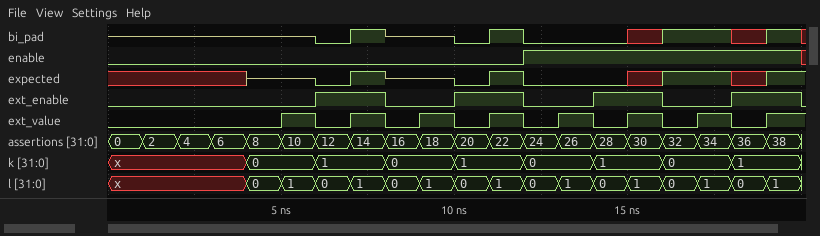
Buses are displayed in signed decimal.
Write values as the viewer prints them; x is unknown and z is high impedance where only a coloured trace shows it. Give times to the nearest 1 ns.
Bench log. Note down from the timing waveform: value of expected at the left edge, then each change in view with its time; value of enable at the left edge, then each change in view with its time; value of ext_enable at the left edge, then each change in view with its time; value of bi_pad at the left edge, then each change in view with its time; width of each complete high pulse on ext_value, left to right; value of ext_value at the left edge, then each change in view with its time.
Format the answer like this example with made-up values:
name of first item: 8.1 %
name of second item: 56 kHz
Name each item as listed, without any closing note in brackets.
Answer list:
value of expected at the left edge, then each change in view with its time: x, z at 4 ns, 0 at 6 ns, 1 at 7 ns, z at 8 ns, 0 at 10 ns, 1 at 11 ns, 0 at 12 ns, x at 15 ns, 1 at 16 ns, x at 18 ns, 1 at 19 ns
value of enable at the left edge, then each change in view with its time: 0, 1 at 12 ns, x at 20 ns
value of ext_enable at the left edge, then each change in view with its time: 0, 1 at 6 ns, 0 at 8 ns, 1 at 10 ns, 0 at 12 ns, 1 at 14 ns, 0 at 16 ns, 1 at 18 ns, 0 at 20 ns
value of bi_pad at the left edge, then each change in view with its time: z, 0 at 6 ns, 1 at 7 ns, z at 8 ns, 0 at 10 ns, 1 at 11 ns, 0 at 12 ns, x at 15 ns, 1 at 16 ns, x at 18 ns, 1 at 19 ns, x at 20 ns
width of each complete high pulse on ext_value, left to right: 1 ns, 1 ns, 1 ns, 1 ns, 1 ns, 1 ns, 1 ns
value of ext_value at the left edge, then each change in view with its time: 0, 1 at 5 ns, 0 at 6 ns, 1 at 7 ns, 0 at 8 ns, 1 at 9 ns, 0 at 10 ns, 1 at 11 ns, 0 at 12 ns, 1 at 13 ns, 0 at 14 ns, 1 at 15 ns, 0 at 16 ns, 1 at 17 ns, 0 at 18 ns, 1 at 19 ns
